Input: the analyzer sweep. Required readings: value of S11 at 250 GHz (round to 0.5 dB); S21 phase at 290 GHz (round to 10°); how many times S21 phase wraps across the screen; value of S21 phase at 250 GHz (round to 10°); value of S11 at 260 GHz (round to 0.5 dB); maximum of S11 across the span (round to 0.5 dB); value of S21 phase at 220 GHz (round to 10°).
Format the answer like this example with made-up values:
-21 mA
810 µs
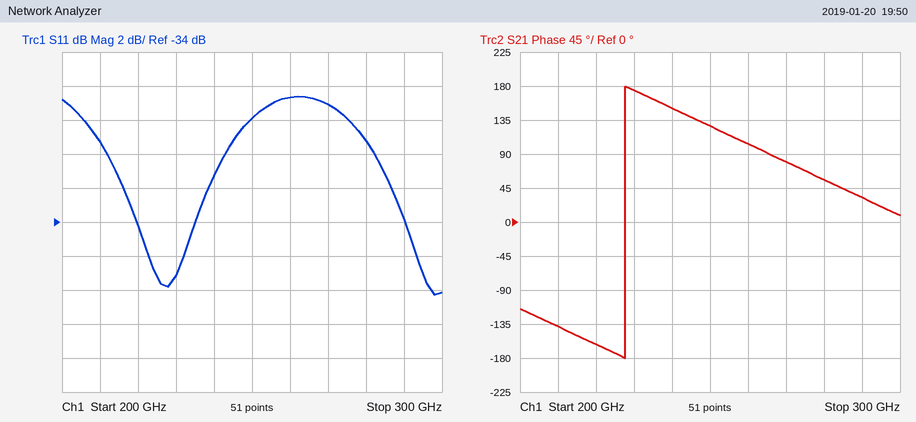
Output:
-28.0 dB
30°
1
130°
-26.5 dB
-26.5 dB
-160°
